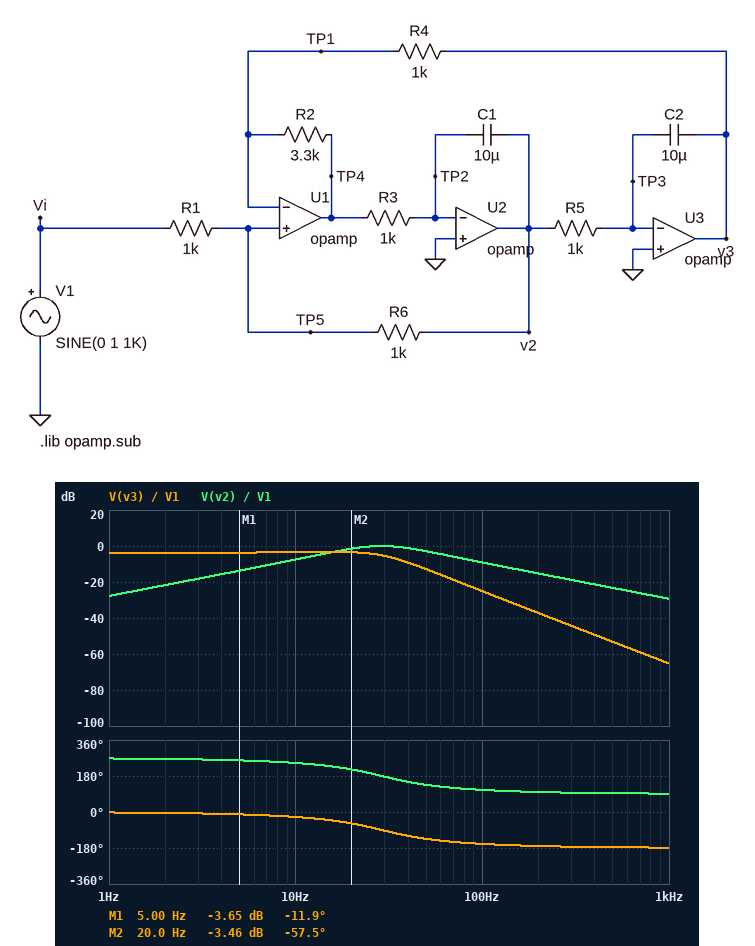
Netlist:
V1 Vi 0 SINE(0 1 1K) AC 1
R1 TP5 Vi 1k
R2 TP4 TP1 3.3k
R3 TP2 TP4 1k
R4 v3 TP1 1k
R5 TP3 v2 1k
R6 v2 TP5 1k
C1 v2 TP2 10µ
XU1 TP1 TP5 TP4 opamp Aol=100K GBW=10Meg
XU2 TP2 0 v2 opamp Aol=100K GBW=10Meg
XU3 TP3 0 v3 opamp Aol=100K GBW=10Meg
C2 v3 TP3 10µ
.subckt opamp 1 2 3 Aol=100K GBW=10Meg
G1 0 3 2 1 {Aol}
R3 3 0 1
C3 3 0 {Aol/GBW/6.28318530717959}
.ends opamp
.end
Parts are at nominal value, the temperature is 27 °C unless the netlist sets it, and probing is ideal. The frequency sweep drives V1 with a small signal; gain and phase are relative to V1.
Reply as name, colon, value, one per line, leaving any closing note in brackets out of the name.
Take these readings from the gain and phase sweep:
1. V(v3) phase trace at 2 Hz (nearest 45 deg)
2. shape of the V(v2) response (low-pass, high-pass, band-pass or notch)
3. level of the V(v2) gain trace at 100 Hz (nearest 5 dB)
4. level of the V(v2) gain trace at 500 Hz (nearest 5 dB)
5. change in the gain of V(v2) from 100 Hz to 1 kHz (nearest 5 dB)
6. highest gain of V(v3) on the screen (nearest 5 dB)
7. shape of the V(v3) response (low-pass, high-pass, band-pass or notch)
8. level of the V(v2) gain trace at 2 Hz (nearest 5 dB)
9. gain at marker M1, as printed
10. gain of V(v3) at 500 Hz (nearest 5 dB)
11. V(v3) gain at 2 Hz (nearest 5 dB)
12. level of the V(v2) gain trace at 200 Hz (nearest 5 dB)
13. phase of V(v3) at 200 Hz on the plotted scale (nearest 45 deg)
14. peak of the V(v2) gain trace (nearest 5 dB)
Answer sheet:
V(v3) phase trace at 2 Hz: 0 deg
shape of the V(v2) response: band-pass
level of the V(v2) gain trace at 100 Hz: -10 dB
level of the V(v2) gain trace at 500 Hz: -25 dB
change in the gain of V(v2) from 100 Hz to 1 kHz: -20 dB
highest gain of V(v3) on the screen: -5 dB
shape of the V(v3) response: low-pass
level of the V(v2) gain trace at 2 Hz: -20 dB
gain at marker M1, as printed: -3.65 dB
gain of V(v3) at 500 Hz: -55 dB
V(v3) gain at 2 Hz: -5 dB
level of the V(v2) gain trace at 200 Hz: -15 dB
phase of V(v3) at 200 Hz on the plotted scale: -180 deg
peak of the V(v2) gain trace: 0 dB
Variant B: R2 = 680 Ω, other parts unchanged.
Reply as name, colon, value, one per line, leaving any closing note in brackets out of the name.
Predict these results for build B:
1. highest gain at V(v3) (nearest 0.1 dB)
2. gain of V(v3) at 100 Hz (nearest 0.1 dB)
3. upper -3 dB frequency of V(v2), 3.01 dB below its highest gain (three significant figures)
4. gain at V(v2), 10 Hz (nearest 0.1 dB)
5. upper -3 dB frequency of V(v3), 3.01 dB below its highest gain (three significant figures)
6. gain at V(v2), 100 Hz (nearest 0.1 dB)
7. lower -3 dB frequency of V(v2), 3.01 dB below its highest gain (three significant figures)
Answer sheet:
highest gain at V(v3): 3.0 dB
gain of V(v3) at 100 Hz: -33.4 dB
upper -3 dB frequency of V(v2), 3.01 dB below its highest gain: 21.4 Hz
gain at V(v2), 10 Hz: -1.1 dB
upper -3 dB frequency of V(v3), 3.01 dB below its highest gain: 15.3 Hz
gain at V(v2), 100 Hz: -17.4 dB
lower -3 dB frequency of V(v2), 3.01 dB below its highest gain: 8.04 Hz
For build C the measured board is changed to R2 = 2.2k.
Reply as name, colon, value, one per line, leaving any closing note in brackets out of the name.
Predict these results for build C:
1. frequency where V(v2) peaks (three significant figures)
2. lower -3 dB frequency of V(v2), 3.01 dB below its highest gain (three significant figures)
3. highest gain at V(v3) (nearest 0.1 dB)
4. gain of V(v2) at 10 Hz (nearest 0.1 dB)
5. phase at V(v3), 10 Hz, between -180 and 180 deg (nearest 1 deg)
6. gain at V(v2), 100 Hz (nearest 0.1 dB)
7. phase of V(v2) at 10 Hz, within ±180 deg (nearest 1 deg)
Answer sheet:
frequency where V(v2) peaks: 23.6 Hz
lower -3 dB frequency of V(v2), 3.01 dB below its highest gain: 14.1 Hz
highest gain at V(v3): -1.9 dB
gain of V(v2) at 10 Hz: -6.3 dB
phase at V(v3), 10 Hz, between -180 and 180 deg: -29 deg
gain at V(v2), 100 Hz: -11.7 dB
phase of V(v2) at 10 Hz, within ±180 deg: -119 deg
